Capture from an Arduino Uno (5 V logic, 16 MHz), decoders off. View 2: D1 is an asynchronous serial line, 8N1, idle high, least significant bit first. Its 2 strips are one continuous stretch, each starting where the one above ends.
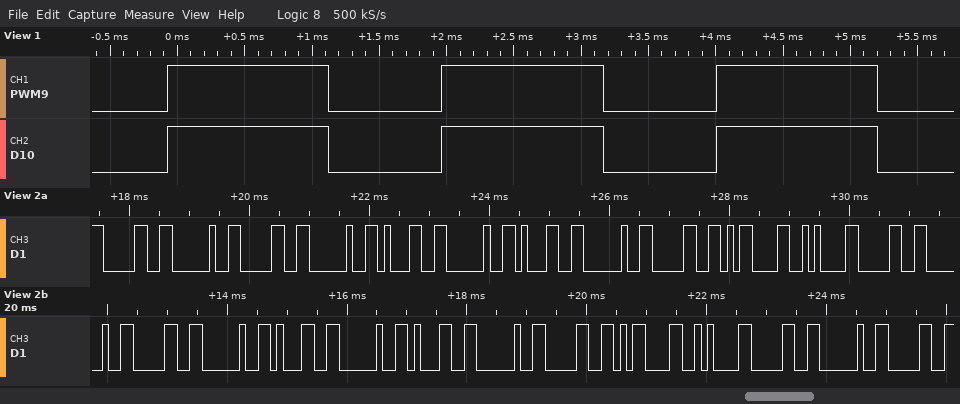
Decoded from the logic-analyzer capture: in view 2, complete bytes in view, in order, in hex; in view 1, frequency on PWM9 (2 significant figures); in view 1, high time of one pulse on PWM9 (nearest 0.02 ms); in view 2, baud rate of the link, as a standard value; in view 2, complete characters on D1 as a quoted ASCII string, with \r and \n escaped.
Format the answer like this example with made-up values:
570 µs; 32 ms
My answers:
0x30 0x20 0x30 0x20 0x31 0x20 0x31 0x20 0x30 0x0D 0x0A 0x30 0x20 0x30 0x20 0x31 0x20 0x31 0x20 0x30 0x0D 0x0A 0x30 0x20 0x30; 490 Hz; 1.20 ms; 9600 baud; "0 0 1 1 0\r\n0 0 1 1 0\r\n0 0"
